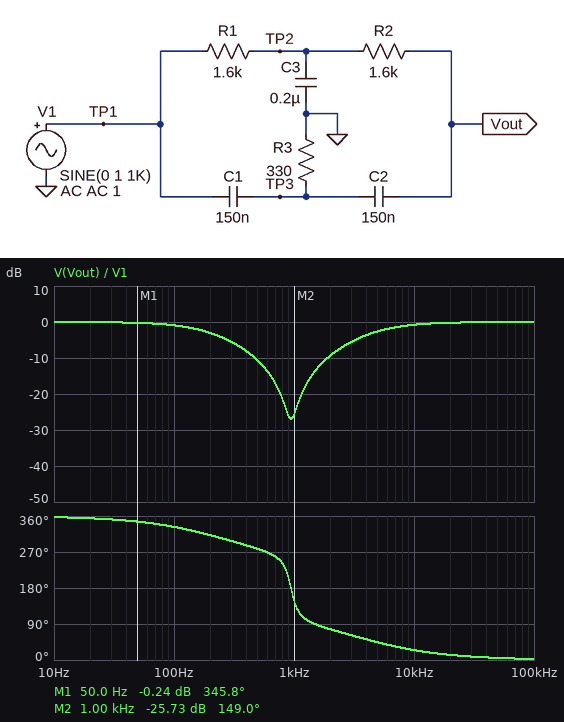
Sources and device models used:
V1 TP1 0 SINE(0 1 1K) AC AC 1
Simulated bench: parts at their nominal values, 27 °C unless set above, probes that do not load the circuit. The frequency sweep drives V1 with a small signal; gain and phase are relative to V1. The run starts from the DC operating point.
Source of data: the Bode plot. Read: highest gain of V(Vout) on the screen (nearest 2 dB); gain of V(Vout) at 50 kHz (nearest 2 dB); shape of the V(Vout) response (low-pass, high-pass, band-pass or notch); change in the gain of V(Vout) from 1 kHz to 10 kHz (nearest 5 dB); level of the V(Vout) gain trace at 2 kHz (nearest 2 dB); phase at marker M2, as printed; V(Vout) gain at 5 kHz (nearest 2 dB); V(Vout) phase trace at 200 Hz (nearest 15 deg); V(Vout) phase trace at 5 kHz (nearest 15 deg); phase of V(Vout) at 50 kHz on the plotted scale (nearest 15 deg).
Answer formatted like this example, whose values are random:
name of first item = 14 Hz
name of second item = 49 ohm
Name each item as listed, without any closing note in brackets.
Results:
highest gain of V(Vout) on the screen = 0 dB
gain of V(Vout) at 50 kHz = 0 dB
shape of the V(Vout) response = notch
change in the gain of V(Vout) from 1 kHz to 10 kHz = 25 dB
level of the V(Vout) gain trace at 2 kHz = -10 dB
phase at marker M2, as printed = 149.0 deg
V(Vout) gain at 5 kHz = -2 dB
V(Vout) phase trace at 200 Hz = 315 deg
V(Vout) phase trace at 5 kHz = 45 deg
phase of V(Vout) at 50 kHz on the plotted scale = 0 deg
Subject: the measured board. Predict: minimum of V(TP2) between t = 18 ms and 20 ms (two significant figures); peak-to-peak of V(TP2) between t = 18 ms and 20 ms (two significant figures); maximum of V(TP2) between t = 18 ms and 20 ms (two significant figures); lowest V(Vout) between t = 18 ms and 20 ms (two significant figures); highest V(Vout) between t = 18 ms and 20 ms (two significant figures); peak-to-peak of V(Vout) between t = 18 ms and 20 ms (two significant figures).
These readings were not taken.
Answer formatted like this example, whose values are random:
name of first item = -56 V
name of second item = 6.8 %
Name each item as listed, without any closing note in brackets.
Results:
minimum of V(TP2) between t = 18 ms and 20 ms = -340 mV
peak-to-peak of V(TP2) between t = 18 ms and 20 ms = 670 mV
maximum of V(TP2) between t = 18 ms and 20 ms = 340 mV
lowest V(Vout) between t = 18 ms and 20 ms = -52 mV
highest V(Vout) between t = 18 ms and 20 ms = 52 mV
peak-to-peak of V(Vout) between t = 18 ms and 20 ms = 100 mV
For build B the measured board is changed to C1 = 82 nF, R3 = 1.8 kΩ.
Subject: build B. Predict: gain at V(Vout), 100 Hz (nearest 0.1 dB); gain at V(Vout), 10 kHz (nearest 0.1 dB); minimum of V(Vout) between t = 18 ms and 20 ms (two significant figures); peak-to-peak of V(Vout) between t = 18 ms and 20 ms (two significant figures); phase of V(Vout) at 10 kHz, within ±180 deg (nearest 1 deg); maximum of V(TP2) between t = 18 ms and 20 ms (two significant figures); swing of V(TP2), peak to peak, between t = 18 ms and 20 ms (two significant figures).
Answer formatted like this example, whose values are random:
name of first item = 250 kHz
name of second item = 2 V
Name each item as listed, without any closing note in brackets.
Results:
gain at V(Vout), 100 Hz = -1.3 dB
gain at V(Vout), 10 kHz = -0.5 dB
minimum of V(Vout) between t = 18 ms and 20 ms = -160 mV
peak-to-peak of V(Vout) between t = 18 ms and 20 ms = 320 mV
phase of V(Vout) at 10 kHz, within ±180 deg = 16 deg
maximum of V(TP2) between t = 18 ms and 20 ms = 400 mV
swing of V(TP2), peak to peak, between t = 18 ms and 20 ms = 800 mV
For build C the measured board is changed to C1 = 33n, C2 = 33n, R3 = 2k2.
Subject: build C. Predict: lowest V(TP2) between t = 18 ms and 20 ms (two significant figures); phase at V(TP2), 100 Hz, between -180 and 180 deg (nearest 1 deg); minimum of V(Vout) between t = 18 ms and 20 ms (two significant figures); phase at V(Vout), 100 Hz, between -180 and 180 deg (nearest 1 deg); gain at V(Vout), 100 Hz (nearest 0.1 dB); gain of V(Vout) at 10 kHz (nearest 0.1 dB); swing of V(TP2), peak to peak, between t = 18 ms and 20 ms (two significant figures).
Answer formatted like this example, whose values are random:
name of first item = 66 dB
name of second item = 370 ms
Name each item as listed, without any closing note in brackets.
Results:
lowest V(TP2) between t = 18 ms and 20 ms = -380 mV
phase at V(TP2), 100 Hz, between -180 and 180 deg = -13 deg
minimum of V(Vout) between t = 18 ms and 20 ms = -250 mV
phase at V(Vout), 100 Hz, between -180 and 180 deg = -15 deg
gain at V(Vout), 100 Hz = -0.3 dB
gain of V(Vout) at 10 kHz = -2.3 dB
swing of V(TP2), peak to peak, between t = 18 ms and 20 ms = 760 mV
